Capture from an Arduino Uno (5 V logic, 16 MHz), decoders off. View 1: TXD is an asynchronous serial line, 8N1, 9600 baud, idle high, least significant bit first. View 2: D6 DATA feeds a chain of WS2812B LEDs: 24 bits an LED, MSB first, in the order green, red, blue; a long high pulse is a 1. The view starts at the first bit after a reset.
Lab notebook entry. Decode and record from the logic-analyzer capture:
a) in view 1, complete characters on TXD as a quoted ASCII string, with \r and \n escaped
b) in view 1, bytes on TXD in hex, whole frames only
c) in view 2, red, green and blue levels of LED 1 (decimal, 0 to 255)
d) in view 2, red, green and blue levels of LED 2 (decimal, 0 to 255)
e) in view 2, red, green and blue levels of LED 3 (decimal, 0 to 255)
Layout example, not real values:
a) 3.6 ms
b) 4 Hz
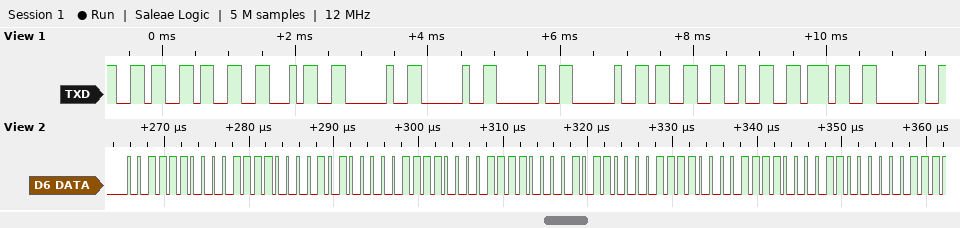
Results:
a) "634    327 "
b) 36 33 34 20 20 20 20 33 32 37 20
c) 60, 60, 40
d) 60, 60, 44
e) 60, 60, 48
